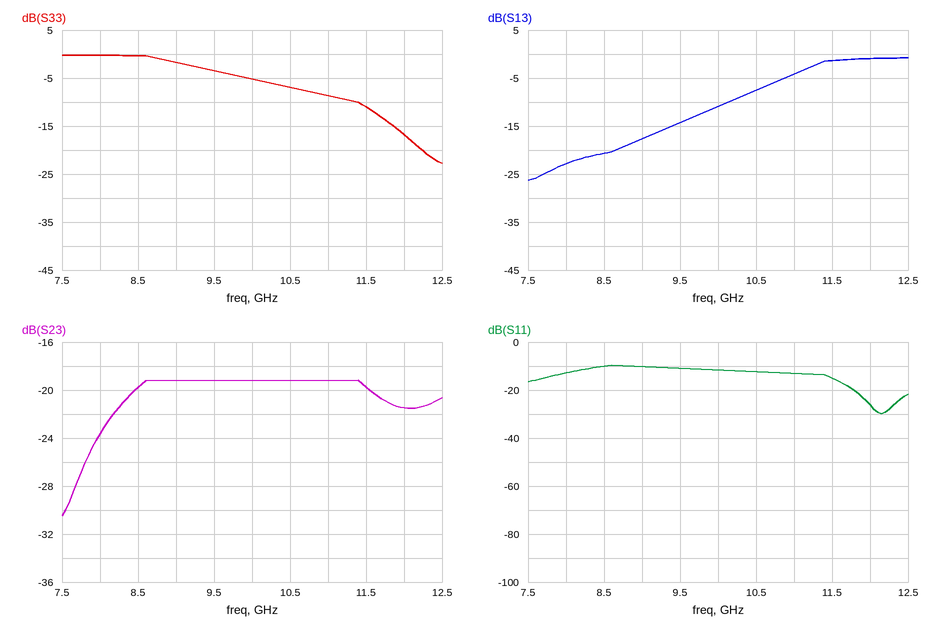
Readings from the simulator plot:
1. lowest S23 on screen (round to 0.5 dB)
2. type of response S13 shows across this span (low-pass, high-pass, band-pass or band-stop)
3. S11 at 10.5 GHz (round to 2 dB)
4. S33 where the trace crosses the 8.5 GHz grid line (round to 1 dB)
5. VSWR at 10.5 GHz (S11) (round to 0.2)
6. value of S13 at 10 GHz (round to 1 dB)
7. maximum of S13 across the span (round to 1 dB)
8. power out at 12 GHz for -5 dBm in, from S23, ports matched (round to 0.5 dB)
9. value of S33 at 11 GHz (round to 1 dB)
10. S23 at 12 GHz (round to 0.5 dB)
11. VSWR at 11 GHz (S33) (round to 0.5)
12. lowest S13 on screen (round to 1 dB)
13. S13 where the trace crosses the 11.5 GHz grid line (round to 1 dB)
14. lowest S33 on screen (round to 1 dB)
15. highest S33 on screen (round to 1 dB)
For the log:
-30.5 dB
high-pass
-12 dB
0 dB
1.6
-11 dB
-1 dB
-26.5 dBm
-9 dB
-21.5 dB
2.0
-26 dB
-1 dB
-23 dB
0 dB
